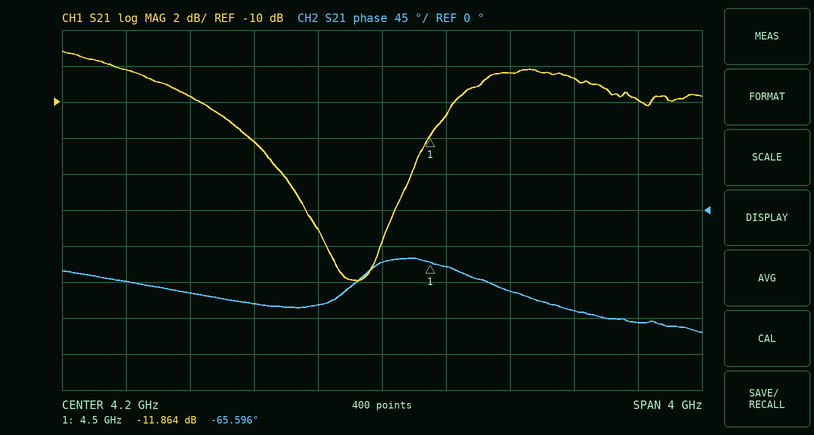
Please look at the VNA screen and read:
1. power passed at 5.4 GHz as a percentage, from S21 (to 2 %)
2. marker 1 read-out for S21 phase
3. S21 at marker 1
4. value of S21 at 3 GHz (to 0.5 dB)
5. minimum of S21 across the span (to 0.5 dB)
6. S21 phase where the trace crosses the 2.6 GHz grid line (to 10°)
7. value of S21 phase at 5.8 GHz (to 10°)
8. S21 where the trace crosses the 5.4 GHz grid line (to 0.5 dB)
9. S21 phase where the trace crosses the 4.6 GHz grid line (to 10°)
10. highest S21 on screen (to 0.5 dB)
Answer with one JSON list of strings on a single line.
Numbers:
["14 %", "-65.596°", "-11.864 dB", "-9.5 dB", "-20.0 dB", "-90°", "-140°", "-8.5 dB", "-70°", "-7.0 dB"]
